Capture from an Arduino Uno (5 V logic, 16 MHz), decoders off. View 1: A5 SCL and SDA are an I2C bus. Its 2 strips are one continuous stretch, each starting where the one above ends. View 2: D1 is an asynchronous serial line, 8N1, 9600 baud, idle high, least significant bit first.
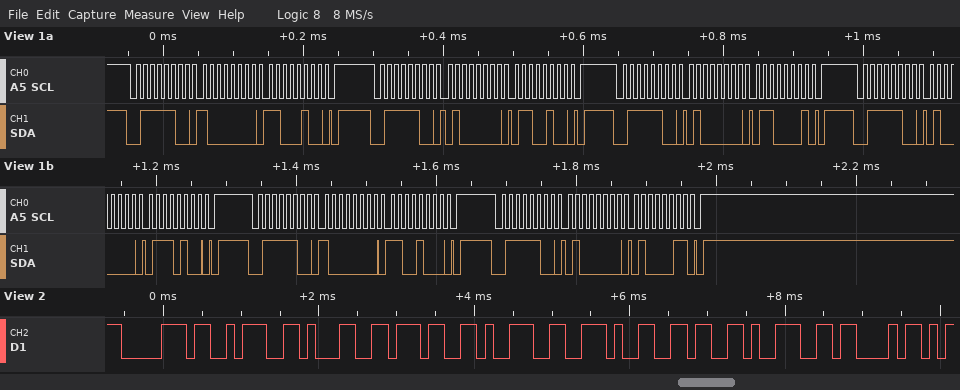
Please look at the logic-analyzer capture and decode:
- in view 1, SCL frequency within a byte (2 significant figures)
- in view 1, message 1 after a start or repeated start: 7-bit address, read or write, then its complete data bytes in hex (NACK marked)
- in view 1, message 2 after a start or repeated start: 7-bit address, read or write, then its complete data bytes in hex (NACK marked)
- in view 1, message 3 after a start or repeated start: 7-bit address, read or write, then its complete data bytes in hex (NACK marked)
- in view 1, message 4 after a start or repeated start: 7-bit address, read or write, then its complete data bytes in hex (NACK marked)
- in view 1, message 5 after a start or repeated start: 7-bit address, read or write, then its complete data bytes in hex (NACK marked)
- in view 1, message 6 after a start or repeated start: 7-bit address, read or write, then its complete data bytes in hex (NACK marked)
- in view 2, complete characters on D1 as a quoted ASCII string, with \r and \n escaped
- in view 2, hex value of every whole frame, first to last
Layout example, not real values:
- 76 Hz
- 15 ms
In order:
- 100 kHz
- 0x3E write: 80 C4
- 0x3E write: 40 64
- 0x3E write: 40 61
- 0x3E write: 40 74
- 0x3E write: 80 C8
- 0x3E write: 40 43
- "p:179.69C"
- 70 3A 31 37 39 2E 36 39 43
